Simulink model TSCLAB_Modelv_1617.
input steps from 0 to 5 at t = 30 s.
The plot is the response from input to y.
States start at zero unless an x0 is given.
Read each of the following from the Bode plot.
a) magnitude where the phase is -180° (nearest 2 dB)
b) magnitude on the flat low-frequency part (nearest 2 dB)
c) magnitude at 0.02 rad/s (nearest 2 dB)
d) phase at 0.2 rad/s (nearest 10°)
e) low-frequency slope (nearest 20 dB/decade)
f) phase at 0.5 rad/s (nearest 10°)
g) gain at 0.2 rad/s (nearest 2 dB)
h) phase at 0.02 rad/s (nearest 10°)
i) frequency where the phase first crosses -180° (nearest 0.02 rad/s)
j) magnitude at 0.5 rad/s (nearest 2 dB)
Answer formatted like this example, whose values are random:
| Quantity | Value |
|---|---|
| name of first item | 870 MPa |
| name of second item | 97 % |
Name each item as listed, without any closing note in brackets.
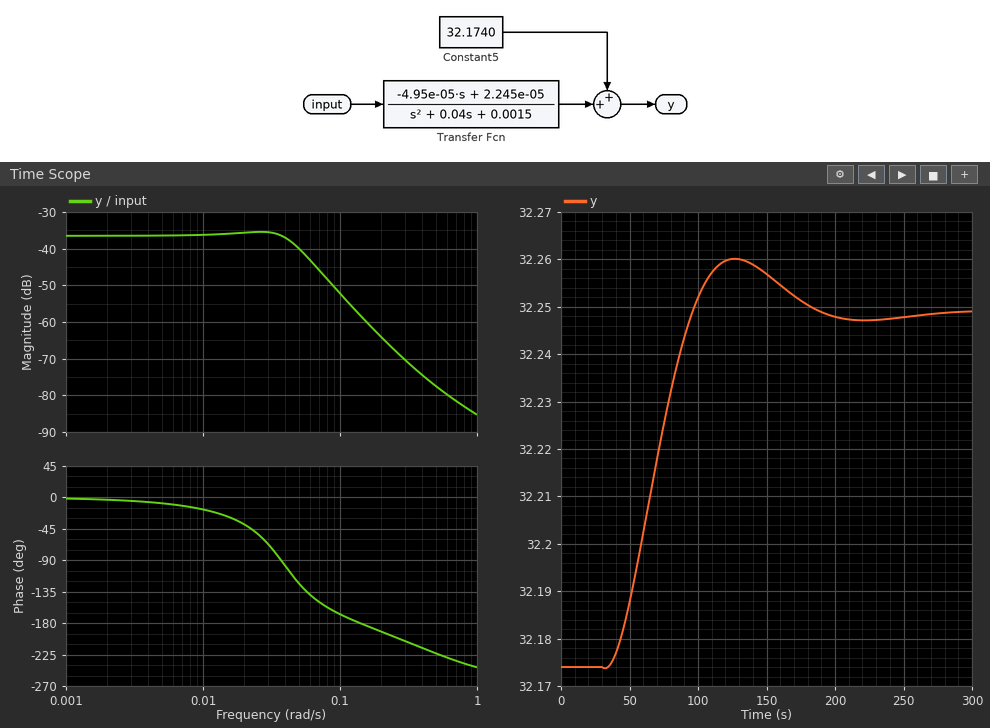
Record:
| Quantity | Value |
|---|---|
| magnitude where the phase is -180° | -58 dB |
| magnitude on the flat low-frequency part | -36 dB |
| magnitude at 0.02 rad/s | -36 dB |
| phase at 0.2 rad/s | -190° |
| low-frequency slope | 0 dB/decade |
| phase at 0.5 rad/s | -220° |
| gain at 0.2 rad/s | -64 dB |
| phase at 0.02 rad/s | -40° |
| frequency where the phase first crosses -180° | 0.14 rad/s |
| magnitude at 0.5 rad/s | -78 dB |
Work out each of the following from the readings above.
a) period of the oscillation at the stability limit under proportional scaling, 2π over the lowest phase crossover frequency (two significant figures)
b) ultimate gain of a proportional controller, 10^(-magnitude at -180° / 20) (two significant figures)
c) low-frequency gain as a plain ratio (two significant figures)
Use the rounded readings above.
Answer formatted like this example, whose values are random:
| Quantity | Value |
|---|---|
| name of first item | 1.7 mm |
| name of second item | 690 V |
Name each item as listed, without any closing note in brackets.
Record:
| Quantity | Value |
|---|---|
| period of the oscillation at the stability limit under proportional scaling, 2π over the lowest phase crossover frequency | 45 s |
| ultimate gain of a proportional controller, 10^(-magnitude at -180° / 20) | 790 |
| low-frequency gain as a plain ratio | 0.016 |
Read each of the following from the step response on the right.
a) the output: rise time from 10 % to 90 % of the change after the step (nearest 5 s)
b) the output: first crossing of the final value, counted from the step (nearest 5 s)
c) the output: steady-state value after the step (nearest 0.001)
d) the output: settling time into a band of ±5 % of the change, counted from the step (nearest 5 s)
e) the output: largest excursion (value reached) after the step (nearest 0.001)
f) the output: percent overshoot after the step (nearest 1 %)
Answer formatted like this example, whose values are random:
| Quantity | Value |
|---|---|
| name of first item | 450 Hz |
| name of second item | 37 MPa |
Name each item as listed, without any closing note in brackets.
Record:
| Quantity | Value |
|---|---|
| the output: rise time from 10 % to 90 % of the change after the step | 45 s |
| the output: first crossing of the final value, counted from the step | 65 s |
| the output: steady-state value after the step | 32.249 |
| the output: settling time into a band of ±5 % of the change, counted from the step | 140 s |
| the output: largest excursion (value reached) after the step | 32.260 |
| the output: percent overshoot after the step | 15 % |
